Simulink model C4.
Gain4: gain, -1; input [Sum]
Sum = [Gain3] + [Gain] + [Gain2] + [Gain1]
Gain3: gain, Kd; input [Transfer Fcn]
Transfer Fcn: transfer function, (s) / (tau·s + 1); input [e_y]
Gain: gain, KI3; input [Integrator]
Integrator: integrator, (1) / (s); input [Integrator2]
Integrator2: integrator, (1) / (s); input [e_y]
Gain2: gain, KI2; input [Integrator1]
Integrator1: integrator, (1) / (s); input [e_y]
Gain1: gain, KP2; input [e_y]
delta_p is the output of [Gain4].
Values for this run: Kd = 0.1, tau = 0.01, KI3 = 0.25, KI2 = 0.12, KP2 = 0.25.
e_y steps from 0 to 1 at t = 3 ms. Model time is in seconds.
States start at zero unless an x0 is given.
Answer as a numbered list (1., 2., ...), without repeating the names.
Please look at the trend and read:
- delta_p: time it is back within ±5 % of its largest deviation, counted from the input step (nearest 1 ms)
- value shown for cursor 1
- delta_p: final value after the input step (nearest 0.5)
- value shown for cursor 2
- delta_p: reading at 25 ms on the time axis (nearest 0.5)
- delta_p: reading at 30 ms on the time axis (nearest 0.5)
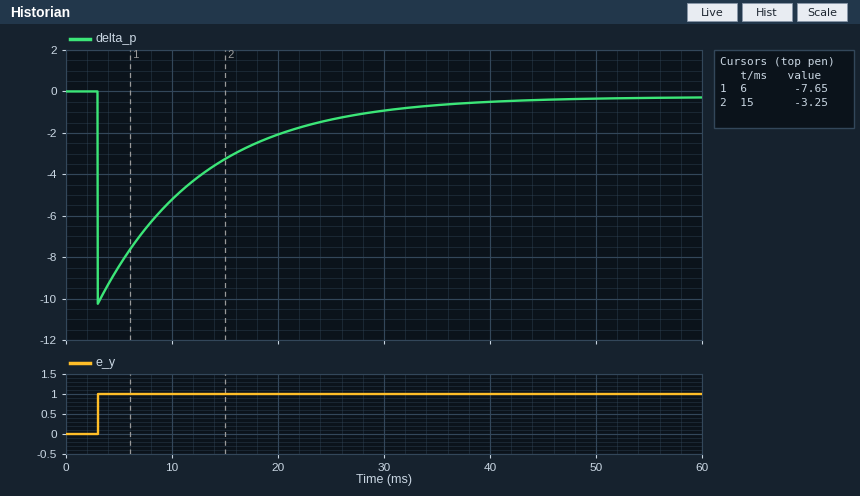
1. 29 ms
2. -7.65
3. -0.5
4. -3.25
5. -1.5
6. -1.0
